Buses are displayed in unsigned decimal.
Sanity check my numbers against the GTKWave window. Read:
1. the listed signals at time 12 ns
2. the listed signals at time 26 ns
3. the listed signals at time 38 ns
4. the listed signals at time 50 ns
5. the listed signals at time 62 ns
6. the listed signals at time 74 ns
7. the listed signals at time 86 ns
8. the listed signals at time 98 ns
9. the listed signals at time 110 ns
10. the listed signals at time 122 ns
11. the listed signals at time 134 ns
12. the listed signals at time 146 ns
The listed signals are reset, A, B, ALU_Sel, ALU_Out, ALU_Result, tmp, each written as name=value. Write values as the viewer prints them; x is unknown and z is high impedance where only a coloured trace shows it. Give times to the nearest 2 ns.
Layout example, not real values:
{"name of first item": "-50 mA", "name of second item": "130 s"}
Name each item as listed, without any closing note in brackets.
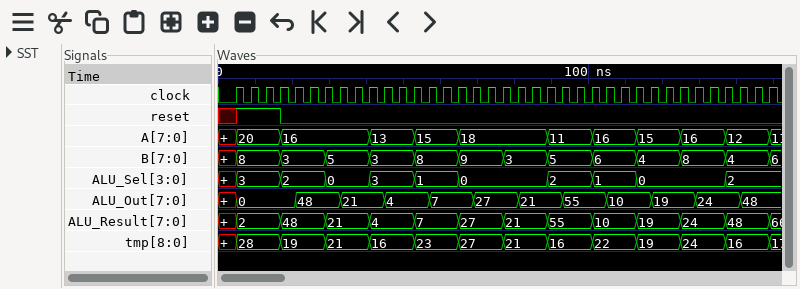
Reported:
{"the listed signals at time 12 ns": "reset=1, A=20, B=8, ALU_Sel=3, ALU_Out=0, ALU_Result=2, tmp=28", "the listed signals at time 26 ns": "reset=0, A=16, B=3, ALU_Sel=2, ALU_Out=48, ALU_Result=48, tmp=19", "the listed signals at time 38 ns": "reset=0, A=16, B=5, ALU_Sel=0, ALU_Out=21, ALU_Result=21, tmp=21", "the listed signals at time 50 ns": "reset=0, A=13, B=3, ALU_Sel=3, ALU_Out=4, ALU_Result=4, tmp=16", "the listed signals at time 62 ns": "reset=0, A=15, B=8, ALU_Sel=1, ALU_Out=7, ALU_Result=7, tmp=23", "the listed signals at time 74 ns": "reset=0, A=18, B=9, ALU_Sel=0, ALU_Out=27, ALU_Result=27, tmp=27", "the listed signals at time 86 ns": "reset=0, A=18, B=3, ALU_Sel=0, ALU_Out=21, ALU_Result=21, tmp=21", "the listed signals at time 98 ns": "reset=0, A=11, B=5, ALU_Sel=2, ALU_Out=55, ALU_Result=55, tmp=16", "the listed signals at time 110 ns": "reset=0, A=16, B=6, ALU_Sel=1, ALU_Out=10, ALU_Result=10, tmp=22", "the listed signals at time 122 ns": "reset=0, A=15, B=4, ALU_Sel=0, ALU_Out=19, ALU_Result=19, tmp=19", "the listed signals at time 134 ns": "reset=0, A=16, B=8, ALU_Sel=0, ALU_Out=24, ALU_Result=24, tmp=24", "the listed signals at time 146 ns": "reset=0, A=12, B=4, ALU_Sel=2, ALU_Out=48, ALU_Result=48, tmp=16"}
